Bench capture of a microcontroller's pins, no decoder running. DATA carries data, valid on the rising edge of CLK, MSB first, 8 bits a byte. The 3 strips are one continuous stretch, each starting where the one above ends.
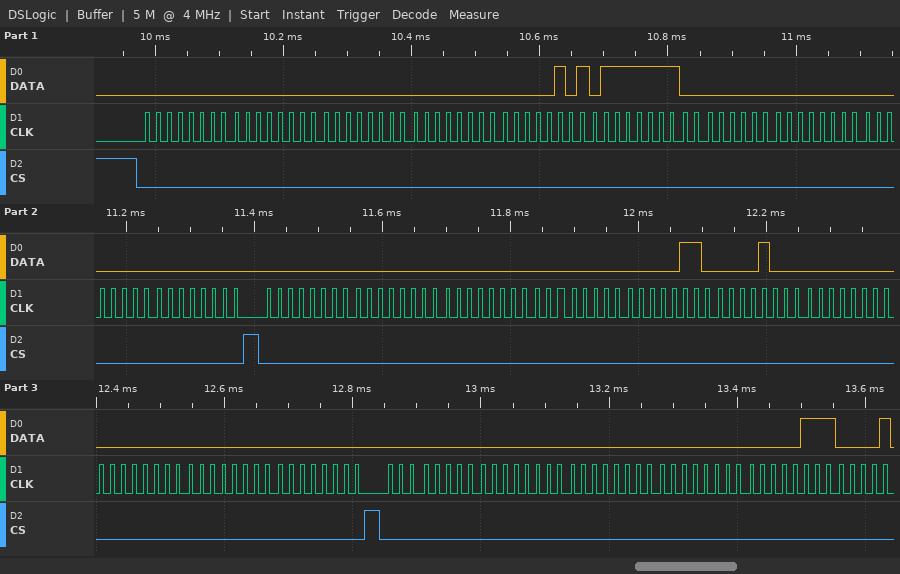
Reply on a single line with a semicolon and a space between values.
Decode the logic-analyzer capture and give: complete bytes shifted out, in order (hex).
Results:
00 00 00 00 05 7F 00 00 00 00 00 00 00 00 06 08 00 00 00 00 00 00 00 00 07
